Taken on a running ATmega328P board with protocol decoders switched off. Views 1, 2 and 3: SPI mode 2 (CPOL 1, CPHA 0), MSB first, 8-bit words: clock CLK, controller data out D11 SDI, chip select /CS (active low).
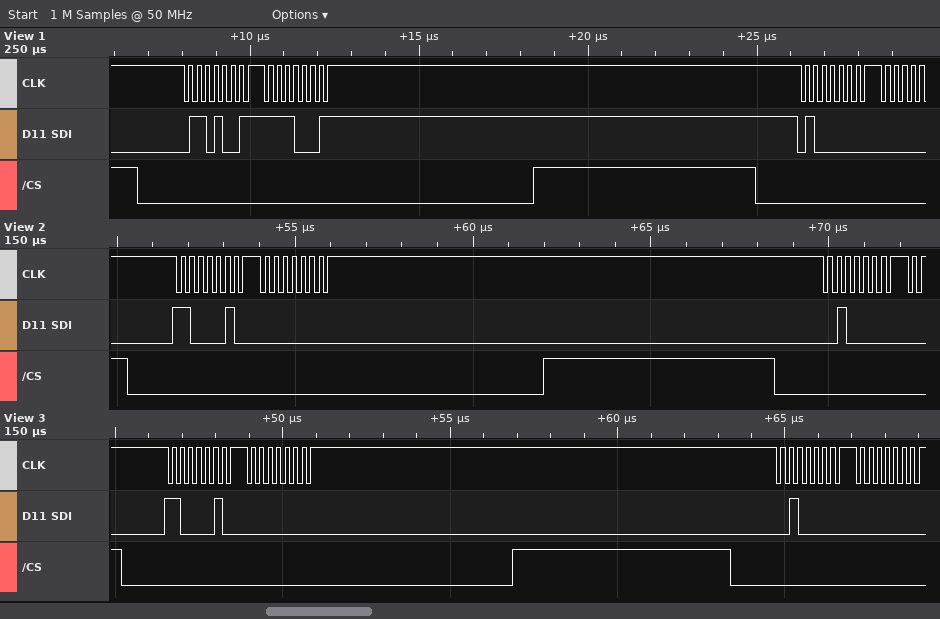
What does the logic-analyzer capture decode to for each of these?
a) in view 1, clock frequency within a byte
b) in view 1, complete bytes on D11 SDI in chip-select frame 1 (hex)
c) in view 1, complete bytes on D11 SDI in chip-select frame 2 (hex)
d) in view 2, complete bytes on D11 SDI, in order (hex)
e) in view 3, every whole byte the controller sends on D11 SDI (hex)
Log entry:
4 MHz
0x69 0xF1
0x40
C2 00 20
C2 00 20 00
